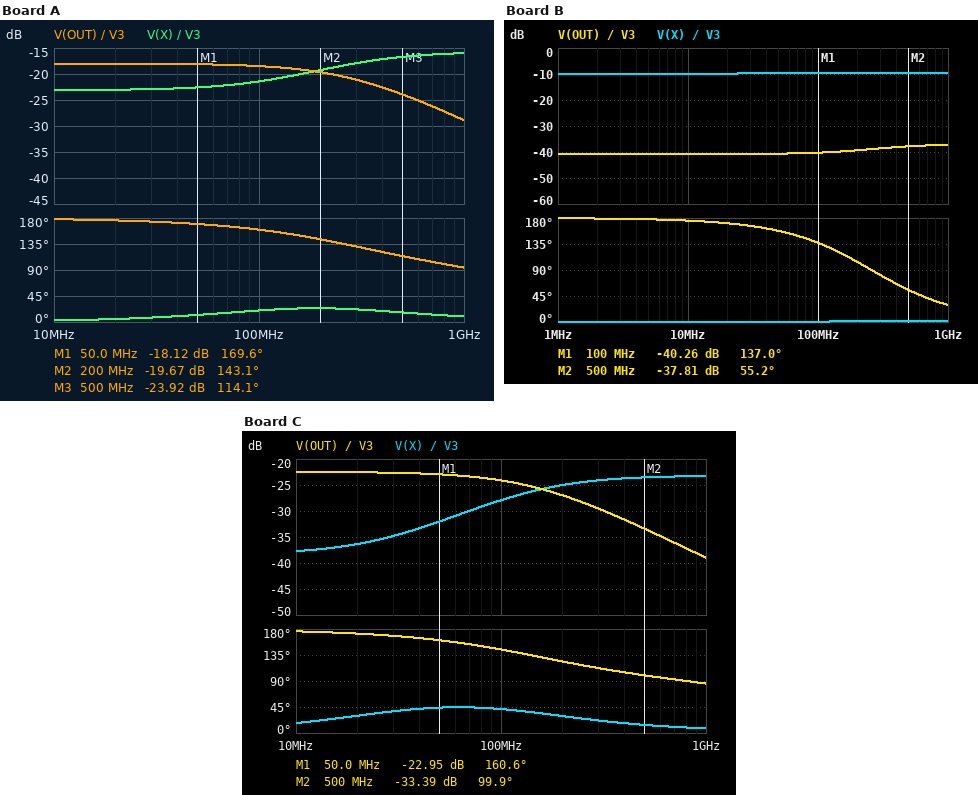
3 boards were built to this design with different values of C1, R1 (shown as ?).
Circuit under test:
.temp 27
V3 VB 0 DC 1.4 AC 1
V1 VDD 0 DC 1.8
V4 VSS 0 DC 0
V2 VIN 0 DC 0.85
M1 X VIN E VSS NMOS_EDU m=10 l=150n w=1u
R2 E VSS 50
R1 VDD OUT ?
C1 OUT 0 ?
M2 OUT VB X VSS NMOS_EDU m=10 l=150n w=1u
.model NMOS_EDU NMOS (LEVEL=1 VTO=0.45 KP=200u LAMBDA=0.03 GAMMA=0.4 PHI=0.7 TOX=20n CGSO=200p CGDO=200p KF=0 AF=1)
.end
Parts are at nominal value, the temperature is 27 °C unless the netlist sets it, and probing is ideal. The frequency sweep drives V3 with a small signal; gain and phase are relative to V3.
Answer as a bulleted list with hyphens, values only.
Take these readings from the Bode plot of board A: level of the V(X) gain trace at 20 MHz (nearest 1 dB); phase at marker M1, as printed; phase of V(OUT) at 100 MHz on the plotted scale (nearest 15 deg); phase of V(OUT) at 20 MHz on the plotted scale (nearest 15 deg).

- -23 dB
- 169.6 deg
- 165 deg
- 180 deg
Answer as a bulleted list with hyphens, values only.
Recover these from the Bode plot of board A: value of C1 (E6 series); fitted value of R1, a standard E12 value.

- 680 fF
- 1.8 kΩ
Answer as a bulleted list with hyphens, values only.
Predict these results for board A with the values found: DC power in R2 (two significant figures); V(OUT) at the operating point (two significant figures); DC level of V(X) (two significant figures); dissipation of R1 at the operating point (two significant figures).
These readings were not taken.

- 30 µW
- 410 mV
- 300 mV
- 1.1 mW
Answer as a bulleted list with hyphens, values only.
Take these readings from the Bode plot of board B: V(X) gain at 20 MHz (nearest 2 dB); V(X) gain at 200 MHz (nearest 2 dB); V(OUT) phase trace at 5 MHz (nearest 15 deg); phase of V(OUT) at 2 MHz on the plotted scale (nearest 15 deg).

- -10 dB
- -10 dB
- 180 deg
- 180 deg
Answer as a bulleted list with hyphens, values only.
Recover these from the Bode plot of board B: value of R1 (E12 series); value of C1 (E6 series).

- 1.5 kΩ
- 330 fF
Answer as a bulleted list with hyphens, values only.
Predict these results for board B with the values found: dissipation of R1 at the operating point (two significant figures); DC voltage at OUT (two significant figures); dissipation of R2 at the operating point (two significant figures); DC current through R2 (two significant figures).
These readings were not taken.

- 1.0 mW
- 570 mV
- 34 µW
- 820 µA
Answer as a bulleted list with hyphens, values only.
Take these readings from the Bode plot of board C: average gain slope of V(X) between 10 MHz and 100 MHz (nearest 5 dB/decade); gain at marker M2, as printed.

- 10 dB/decade
- -33.39 dB
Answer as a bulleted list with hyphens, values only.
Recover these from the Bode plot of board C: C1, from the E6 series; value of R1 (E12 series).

- 2.2 pF
- 2.7 kΩ
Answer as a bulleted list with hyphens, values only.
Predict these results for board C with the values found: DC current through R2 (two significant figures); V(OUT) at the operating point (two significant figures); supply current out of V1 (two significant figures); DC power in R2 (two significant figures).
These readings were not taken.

- 580 µA
- 240 mV
- 580 µA
- 17 µW
